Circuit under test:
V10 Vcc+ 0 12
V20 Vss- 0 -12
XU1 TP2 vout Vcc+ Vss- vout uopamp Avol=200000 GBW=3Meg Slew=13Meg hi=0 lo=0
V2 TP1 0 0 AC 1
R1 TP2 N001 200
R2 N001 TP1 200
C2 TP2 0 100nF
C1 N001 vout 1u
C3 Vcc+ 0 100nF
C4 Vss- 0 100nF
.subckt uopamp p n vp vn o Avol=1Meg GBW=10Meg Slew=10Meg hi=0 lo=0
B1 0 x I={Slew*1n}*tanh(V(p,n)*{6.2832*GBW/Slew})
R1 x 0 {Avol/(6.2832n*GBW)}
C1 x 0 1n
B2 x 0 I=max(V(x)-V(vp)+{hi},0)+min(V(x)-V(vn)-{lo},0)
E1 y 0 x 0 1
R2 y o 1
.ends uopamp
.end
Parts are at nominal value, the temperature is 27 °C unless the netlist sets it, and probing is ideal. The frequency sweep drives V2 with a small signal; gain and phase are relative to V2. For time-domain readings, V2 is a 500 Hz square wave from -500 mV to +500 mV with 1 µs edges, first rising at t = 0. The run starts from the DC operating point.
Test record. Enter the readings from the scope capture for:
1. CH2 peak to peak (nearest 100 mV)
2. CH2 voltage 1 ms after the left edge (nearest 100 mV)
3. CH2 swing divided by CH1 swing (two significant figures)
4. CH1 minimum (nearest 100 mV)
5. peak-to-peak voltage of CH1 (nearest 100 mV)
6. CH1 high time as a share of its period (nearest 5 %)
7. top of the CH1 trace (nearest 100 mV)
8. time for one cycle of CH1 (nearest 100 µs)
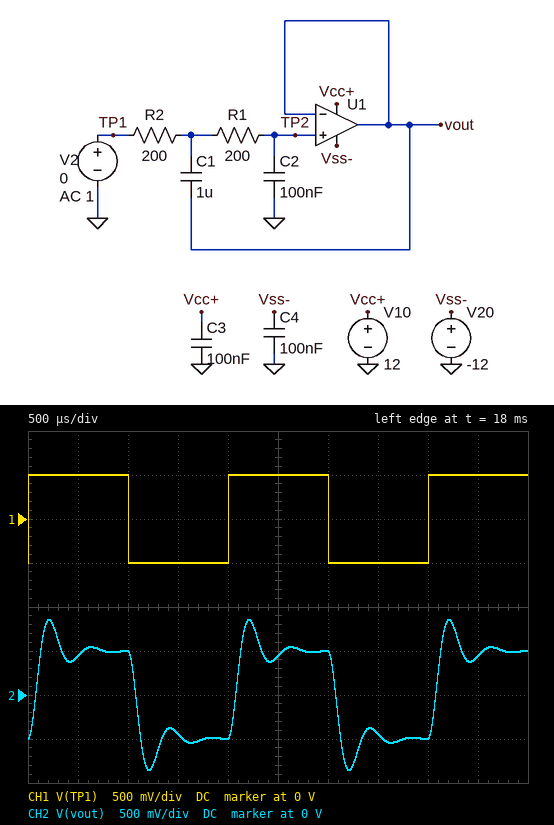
1.7 V
500 mV
1.7
-500 mV
1.0 V
50 %
500 mV
2.0 ms
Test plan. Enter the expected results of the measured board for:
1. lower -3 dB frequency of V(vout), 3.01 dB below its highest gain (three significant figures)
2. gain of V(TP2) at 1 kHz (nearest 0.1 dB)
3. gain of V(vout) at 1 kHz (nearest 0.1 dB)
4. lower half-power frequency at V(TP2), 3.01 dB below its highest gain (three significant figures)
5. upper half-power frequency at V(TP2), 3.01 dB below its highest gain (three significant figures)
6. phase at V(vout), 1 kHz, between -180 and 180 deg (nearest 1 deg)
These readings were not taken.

1.13 kHz
1.1 dB
1.1 dB
1.13 kHz
2.97 kHz
-17 deg
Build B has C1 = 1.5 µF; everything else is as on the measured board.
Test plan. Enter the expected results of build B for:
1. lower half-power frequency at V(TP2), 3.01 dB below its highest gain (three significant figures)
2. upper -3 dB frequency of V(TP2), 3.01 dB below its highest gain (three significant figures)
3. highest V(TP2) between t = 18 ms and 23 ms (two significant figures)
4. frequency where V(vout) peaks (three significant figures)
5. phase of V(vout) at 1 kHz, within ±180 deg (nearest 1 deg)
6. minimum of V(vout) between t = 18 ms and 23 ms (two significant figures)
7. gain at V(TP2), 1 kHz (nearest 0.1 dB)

1.25 kHz
2.40 kHz
920 mV
1.91 kHz
-18 deg
-920 mV
1.9 dB
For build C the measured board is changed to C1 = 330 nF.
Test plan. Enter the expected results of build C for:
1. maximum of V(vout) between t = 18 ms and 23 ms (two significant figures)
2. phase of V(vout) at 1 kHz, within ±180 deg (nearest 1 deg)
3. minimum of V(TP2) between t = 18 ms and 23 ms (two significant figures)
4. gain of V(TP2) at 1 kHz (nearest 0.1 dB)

630 mV
-15 deg
-630 mV
0.2 dB
